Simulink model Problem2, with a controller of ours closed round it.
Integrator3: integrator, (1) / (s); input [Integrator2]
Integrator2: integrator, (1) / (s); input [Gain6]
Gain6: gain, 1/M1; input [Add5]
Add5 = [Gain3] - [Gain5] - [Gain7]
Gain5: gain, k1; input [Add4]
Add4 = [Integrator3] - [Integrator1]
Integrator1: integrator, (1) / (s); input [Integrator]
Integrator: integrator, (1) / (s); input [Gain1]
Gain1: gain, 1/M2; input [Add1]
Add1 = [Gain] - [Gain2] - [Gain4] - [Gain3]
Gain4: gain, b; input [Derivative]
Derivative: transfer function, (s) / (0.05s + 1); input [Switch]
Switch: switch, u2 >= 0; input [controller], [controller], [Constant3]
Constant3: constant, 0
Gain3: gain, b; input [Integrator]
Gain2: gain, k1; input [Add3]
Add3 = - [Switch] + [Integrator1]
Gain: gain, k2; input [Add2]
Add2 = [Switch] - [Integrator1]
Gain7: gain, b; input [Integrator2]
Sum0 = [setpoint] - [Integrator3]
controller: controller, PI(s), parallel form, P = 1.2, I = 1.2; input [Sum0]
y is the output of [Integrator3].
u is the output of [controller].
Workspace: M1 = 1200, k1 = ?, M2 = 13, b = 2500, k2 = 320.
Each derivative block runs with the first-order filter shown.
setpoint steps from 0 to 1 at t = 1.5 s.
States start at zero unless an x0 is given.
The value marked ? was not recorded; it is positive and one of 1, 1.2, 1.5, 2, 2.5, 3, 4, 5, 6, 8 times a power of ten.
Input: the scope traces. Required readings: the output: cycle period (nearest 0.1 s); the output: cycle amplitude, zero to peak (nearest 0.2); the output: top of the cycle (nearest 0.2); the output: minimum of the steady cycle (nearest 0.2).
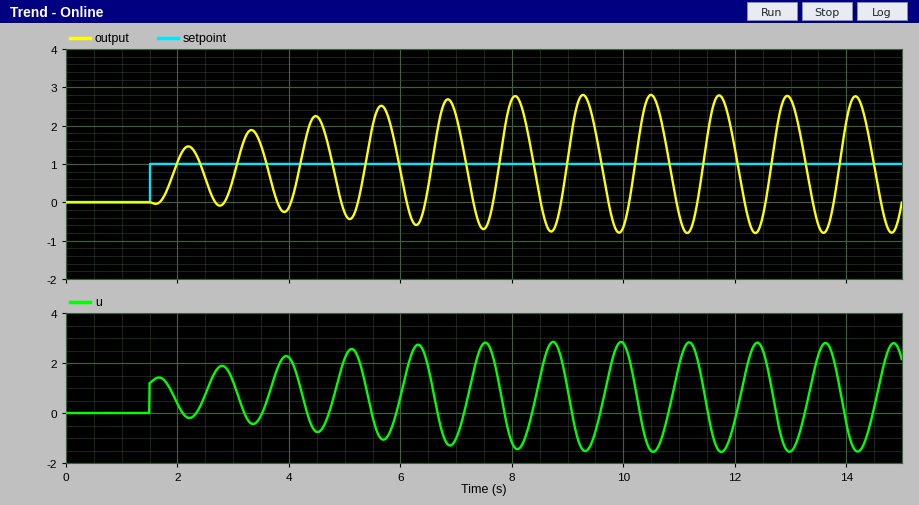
1.2 s
1.8
2.8
-0.8
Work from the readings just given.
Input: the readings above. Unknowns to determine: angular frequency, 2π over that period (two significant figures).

5.2 rad/s
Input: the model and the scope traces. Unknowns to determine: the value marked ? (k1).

20000
